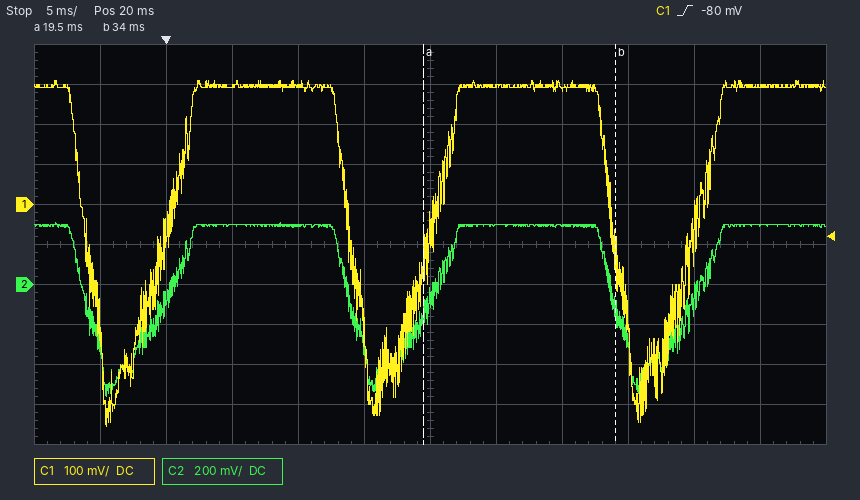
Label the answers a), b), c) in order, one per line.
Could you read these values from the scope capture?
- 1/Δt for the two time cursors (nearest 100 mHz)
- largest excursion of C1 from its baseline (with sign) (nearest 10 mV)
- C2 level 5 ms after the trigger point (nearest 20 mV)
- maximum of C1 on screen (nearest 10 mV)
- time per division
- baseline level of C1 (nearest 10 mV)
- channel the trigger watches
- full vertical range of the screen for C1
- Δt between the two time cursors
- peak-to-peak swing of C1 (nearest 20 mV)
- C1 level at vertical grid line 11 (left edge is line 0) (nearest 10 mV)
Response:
a) 69.0 Hz
b) -850 mV
c) 300 mV
d) 310 mV
e) 5 ms
f) 300 mV
g) C1
h) 1 V
i) 14.5 ms
j) 860 mV
k) 300 mV
